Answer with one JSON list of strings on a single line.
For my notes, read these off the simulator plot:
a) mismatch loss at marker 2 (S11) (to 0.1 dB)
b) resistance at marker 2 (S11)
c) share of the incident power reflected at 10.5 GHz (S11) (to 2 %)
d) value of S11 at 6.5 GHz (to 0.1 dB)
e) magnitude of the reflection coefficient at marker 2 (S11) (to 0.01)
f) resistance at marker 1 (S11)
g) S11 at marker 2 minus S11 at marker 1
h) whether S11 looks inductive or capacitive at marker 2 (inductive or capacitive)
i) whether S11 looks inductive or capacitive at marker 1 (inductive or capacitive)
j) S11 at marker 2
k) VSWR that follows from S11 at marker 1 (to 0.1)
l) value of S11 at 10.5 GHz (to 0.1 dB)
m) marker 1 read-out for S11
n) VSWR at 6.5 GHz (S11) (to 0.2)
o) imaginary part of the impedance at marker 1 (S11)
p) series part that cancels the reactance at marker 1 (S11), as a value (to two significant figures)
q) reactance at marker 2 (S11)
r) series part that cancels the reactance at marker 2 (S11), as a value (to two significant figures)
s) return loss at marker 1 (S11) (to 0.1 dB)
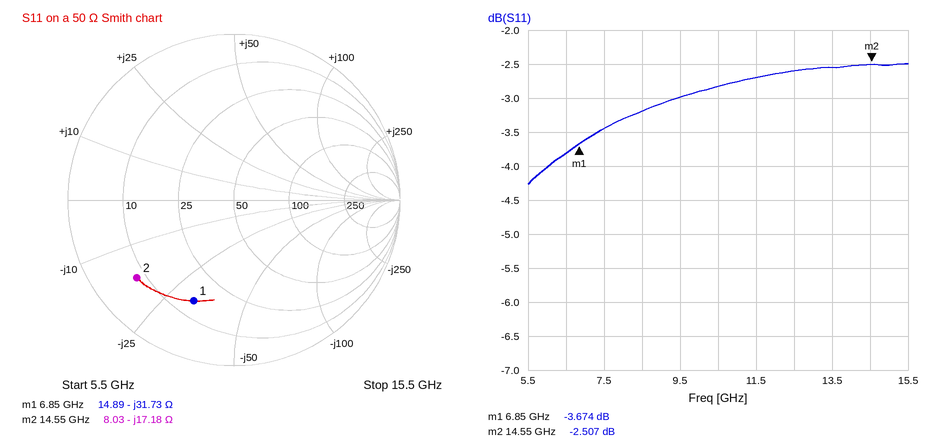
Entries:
["3.6 dB", "8.03 Ω", "52 %", "-3.8 dB", "0.75", "14.89 Ω", "1.167 dB", "capacitive", "capacitive", "-2.507 dB", "4.8", "-2.8 dB", "-3.674 dB", "4.6", "-31.73 Ω", "740 pH", "-17.18 Ω", "190 pH", "3.7 dB"]
